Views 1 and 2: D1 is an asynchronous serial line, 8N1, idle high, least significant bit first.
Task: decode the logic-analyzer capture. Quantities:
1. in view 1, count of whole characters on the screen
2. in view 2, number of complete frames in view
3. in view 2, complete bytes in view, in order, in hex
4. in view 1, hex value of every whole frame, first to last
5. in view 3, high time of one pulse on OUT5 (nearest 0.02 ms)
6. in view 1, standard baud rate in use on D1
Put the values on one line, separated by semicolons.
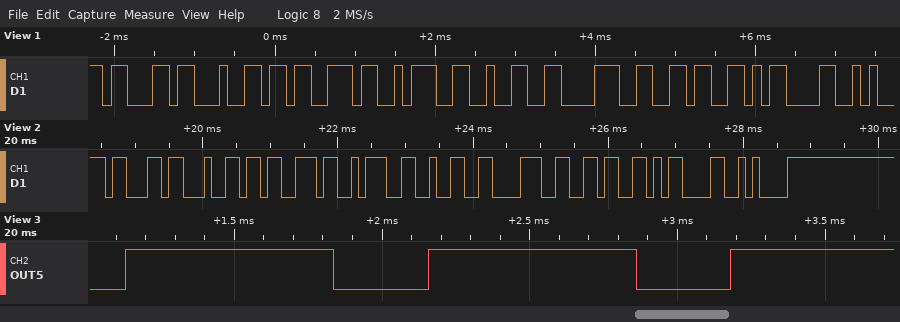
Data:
8; 9; 63 64 73 3A 32 38 36 0D 0A; 63 64 73 3A 32 38 36 0D; 0.70 ms; 9600 baud
